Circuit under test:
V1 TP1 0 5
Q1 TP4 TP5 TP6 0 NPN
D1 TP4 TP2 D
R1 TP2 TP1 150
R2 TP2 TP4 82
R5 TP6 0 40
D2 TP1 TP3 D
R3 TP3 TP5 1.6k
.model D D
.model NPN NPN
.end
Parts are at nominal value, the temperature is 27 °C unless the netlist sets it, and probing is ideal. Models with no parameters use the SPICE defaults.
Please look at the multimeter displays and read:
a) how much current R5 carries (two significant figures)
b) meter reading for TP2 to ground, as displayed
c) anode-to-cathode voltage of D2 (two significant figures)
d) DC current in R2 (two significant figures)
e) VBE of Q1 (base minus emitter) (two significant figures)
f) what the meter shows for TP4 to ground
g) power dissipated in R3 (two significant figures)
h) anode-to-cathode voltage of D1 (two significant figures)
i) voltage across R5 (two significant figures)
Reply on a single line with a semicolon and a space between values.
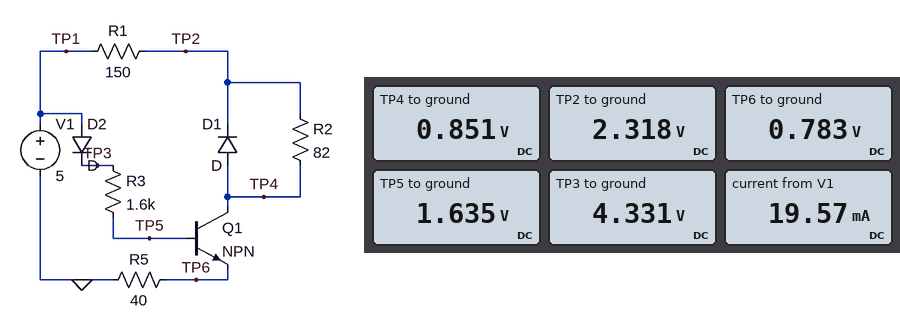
20 mA; 2.318 V; 670 mV; 18 mA; 850 mV; 0.851 V; 4.5 mW; -1.5 V; 780 mV
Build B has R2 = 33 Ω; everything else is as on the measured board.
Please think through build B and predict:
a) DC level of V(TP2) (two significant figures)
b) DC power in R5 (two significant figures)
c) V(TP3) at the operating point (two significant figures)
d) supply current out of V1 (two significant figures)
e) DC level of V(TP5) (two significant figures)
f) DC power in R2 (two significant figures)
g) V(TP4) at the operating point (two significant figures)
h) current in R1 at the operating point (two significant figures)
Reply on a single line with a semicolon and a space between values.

1.7 V; 22 mW; 4.3 V; 23 mA; 1.8 V; 16 mW; 1.0 V; 22 mA
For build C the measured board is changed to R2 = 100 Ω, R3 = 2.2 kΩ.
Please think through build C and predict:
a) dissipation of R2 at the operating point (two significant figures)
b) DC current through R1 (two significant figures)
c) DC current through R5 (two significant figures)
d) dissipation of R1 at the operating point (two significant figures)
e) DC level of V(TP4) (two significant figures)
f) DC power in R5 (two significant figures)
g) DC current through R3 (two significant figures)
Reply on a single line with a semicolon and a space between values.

28 mW; 17 mA; 18 mA; 42 mW; 800 mV; 13 mW; 1.3 mA
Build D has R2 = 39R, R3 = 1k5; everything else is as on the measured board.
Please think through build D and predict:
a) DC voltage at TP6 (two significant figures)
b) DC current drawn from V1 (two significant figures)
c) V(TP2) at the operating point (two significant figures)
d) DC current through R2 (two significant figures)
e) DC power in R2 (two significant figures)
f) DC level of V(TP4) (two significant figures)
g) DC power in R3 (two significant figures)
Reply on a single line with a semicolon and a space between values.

920 mV; 23 mA; 1.8 V; 21 mA; 18 mW; 990 mV; 4.4 mW
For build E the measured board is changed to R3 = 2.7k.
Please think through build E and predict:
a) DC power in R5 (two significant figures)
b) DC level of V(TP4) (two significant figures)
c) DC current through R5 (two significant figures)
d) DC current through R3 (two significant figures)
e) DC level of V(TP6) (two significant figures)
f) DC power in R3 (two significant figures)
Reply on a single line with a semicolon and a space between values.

14 mW; 840 mV; 19 mA; 1.0 mA; 760 mV; 2.8 mW
